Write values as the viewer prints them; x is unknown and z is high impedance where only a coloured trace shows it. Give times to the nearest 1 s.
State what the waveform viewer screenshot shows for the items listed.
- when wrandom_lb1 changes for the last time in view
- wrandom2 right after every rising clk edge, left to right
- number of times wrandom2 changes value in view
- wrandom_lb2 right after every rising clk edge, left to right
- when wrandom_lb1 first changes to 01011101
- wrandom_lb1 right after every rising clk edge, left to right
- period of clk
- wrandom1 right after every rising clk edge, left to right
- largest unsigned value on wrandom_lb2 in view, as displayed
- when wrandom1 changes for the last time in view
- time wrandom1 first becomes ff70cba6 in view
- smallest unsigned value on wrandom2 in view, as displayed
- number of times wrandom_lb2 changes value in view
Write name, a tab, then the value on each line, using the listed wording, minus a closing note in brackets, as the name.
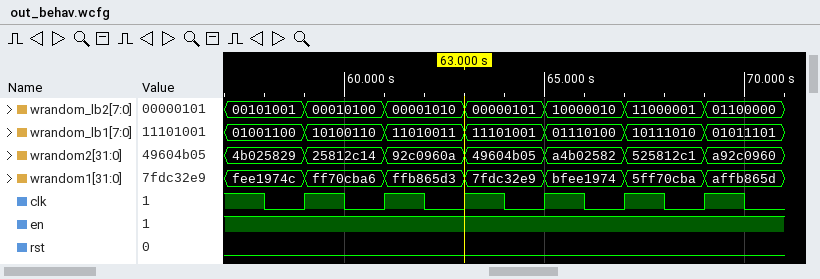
when wrandom_lb1 changes for the last time in view	69 s
wrandom2 right after every rising clk edge, left to right	25812c14, 92c0960a, 49604b05, a4b02582, 525812c1, a92c0960
number of times wrandom2 changes value in view	6
wrandom_lb2 right after every rising clk edge, left to right	00010100, 00001010, 00000101, 10000010, 11000001, 01100000
when wrandom_lb1 first changes to 01011101	69 s
wrandom_lb1 right after every rising clk edge, left to right	10100110, 11010011, 11101001, 01110100, 10111010, 01011101
period of clk	2 s
wrandom1 right after every rising clk edge, left to right	ff70cba6, ffb865d3, 7fdc32e9, bfee1974, 5ff70cba, affb865d
largest unsigned value on wrandom_lb2 in view, as displayed	11000001
when wrandom1 changes for the last time in view	69 s
time wrandom1 first becomes ff70cba6 in view	59 s
smallest unsigned value on wrandom2 in view, as displayed	25812c14
number of times wrandom_lb2 changes value in view	6
